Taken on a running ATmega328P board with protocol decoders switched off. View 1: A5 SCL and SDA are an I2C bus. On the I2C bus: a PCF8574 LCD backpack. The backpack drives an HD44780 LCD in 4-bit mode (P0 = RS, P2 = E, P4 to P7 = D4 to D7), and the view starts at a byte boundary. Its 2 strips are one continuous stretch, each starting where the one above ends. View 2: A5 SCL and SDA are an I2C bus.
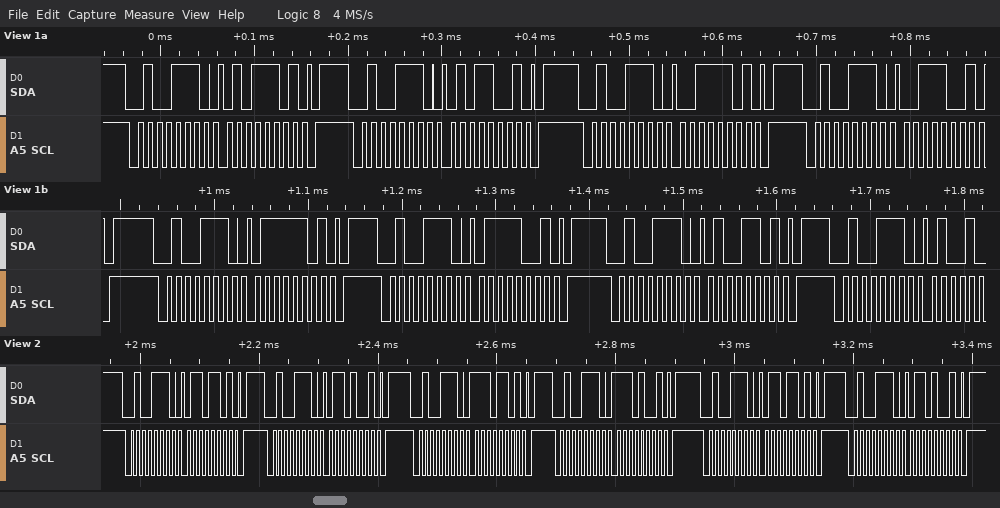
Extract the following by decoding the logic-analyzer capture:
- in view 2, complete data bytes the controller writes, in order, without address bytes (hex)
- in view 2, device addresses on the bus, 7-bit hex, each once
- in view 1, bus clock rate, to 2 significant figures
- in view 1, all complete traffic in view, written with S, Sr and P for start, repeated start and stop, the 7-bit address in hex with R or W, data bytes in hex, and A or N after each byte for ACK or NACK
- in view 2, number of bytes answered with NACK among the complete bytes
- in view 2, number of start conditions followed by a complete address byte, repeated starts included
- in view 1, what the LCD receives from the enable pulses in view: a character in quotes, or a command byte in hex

6D 69 ED E9 6D 69
0x27
100 kHz
S 27W A 5D A P S 27W A 59 A P S 27W A 3D A P S 27W A 39 A P S 27W A 7D A P S 27W A 79 A P S 27W A 4D A P S 27W A
0
6
'S'
